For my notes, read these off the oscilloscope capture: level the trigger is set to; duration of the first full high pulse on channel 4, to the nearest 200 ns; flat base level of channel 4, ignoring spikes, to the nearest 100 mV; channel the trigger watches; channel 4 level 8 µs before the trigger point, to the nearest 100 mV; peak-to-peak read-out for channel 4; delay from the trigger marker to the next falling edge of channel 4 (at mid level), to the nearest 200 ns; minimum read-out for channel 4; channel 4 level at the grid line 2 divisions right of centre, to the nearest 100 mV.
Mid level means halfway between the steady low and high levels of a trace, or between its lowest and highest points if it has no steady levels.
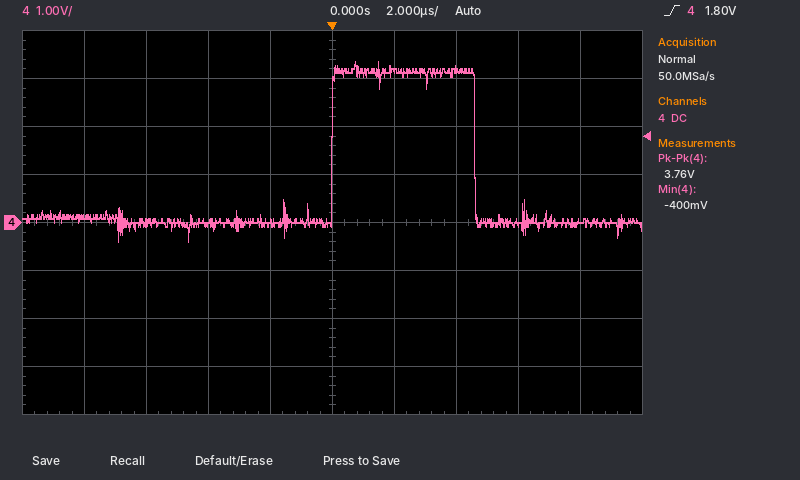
1.80 V
4.6 µs
0.0 V
channel 4
100 mV
3.76 V
4.6 µs
-400 mV
3.2 V
